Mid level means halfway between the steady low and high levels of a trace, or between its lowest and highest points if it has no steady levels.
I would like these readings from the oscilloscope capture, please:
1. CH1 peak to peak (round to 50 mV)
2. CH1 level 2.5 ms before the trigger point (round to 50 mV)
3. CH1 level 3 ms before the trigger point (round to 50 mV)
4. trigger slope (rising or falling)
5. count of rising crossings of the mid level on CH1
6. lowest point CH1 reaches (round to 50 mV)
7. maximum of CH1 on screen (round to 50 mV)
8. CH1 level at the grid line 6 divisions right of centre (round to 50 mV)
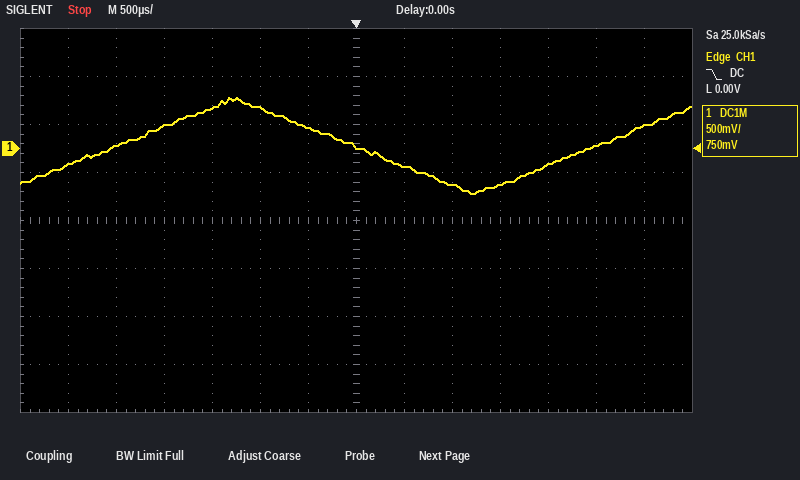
1.00 V
50 mV
-150 mV
falling
2
-450 mV
550 mV
250 mV
